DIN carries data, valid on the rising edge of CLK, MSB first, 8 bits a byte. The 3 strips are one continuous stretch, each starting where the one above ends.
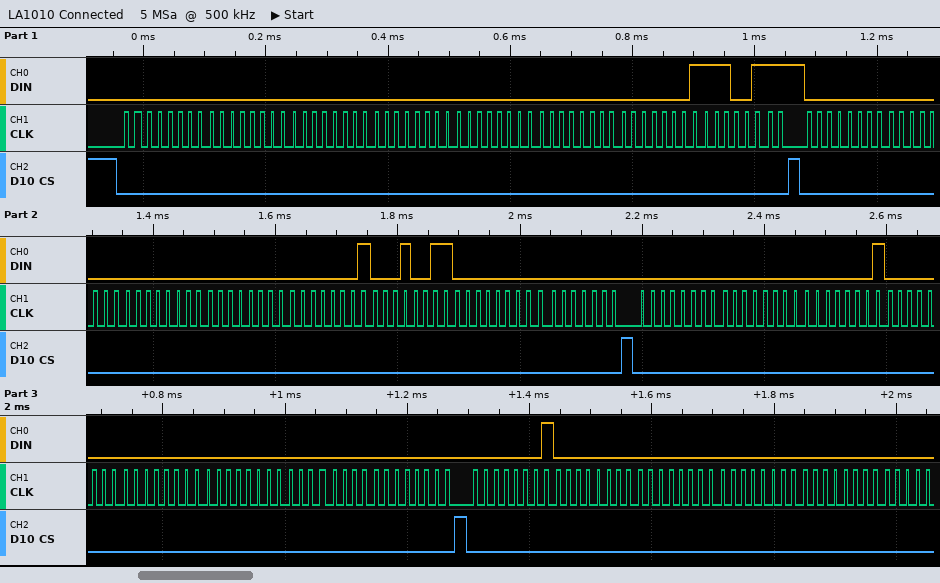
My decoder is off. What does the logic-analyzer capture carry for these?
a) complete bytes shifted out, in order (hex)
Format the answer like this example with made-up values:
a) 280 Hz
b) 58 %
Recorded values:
a) 00 00 00 00 00 00 01 E7 00 00 00 00 01 13 00 00 00 00 01 00 00 00 00 00 01 00 00 00 00
